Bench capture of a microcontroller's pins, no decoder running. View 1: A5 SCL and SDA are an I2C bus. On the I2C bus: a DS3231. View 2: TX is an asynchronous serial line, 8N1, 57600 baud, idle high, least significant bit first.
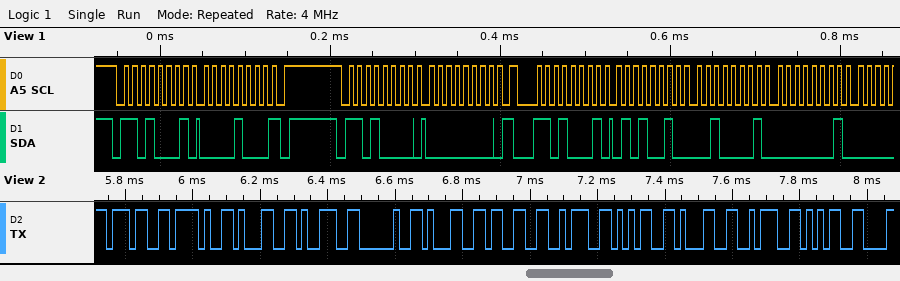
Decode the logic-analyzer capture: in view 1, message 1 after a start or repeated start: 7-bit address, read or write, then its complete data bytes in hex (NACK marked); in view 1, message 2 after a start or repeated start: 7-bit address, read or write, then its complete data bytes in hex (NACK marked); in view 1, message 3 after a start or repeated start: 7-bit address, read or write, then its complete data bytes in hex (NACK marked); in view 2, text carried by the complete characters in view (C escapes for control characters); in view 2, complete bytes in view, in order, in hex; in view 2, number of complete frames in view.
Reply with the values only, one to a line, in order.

0x68 read: 08 NACK
0x68 write: 00
0x68 read: 52 21 01
"7/19 13:51:5"
37 2F 31 39 20 31 33 3A 35 31 3A 35
12
